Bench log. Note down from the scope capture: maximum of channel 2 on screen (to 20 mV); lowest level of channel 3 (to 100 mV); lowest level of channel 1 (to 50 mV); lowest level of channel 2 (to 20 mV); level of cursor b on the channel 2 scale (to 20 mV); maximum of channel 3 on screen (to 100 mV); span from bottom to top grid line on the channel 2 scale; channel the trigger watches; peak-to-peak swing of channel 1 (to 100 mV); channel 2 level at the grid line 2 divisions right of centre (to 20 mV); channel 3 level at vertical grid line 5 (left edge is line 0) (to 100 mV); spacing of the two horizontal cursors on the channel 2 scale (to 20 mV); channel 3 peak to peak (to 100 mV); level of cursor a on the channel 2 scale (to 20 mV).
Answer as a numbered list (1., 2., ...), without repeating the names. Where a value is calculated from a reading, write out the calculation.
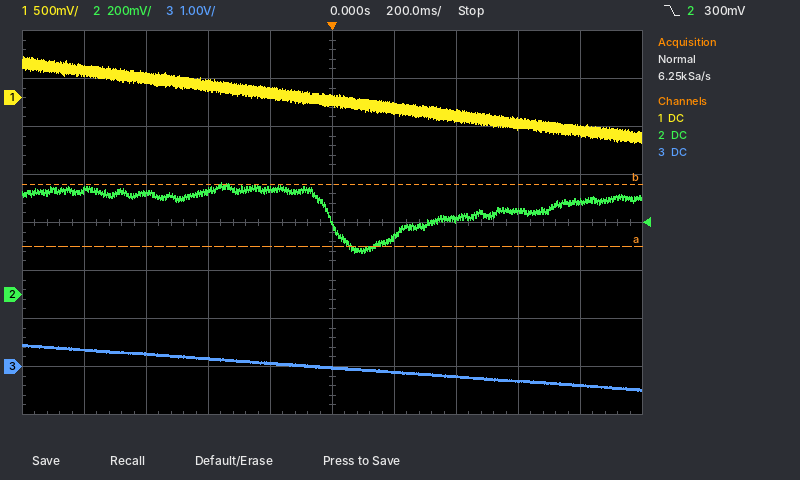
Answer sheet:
1. 460 mV
2. -500 mV
3. -450 mV
4. 180 mV
5. 460 mV
6. 500 mV
7. 1.6 V
8. channel 2
9. 900 mV
10. 320 mV
11. 0.0 V
12. 260 mV
13. 500 mV − (-500 mV) = 1.0 V
14. 200 mV
